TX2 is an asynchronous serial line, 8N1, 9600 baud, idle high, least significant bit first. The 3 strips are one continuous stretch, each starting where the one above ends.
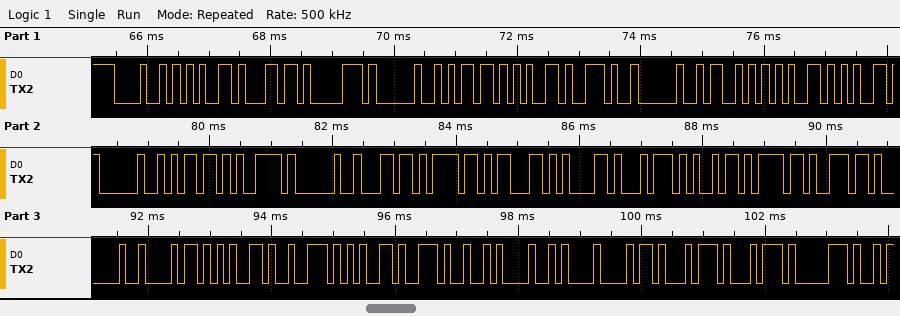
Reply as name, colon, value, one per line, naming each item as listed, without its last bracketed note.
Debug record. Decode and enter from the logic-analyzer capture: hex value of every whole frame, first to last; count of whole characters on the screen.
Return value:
hex value of every whole frame, first to last: 48 65 6C 70 20 6D 65 2E 20 53 65 65 20 6D 79 20 6C 6F 63 61 74 69 6F 6E 20 68 65 72 65 2E 0A 0A 68 74 74 70
count of whole characters on the screen: 36
